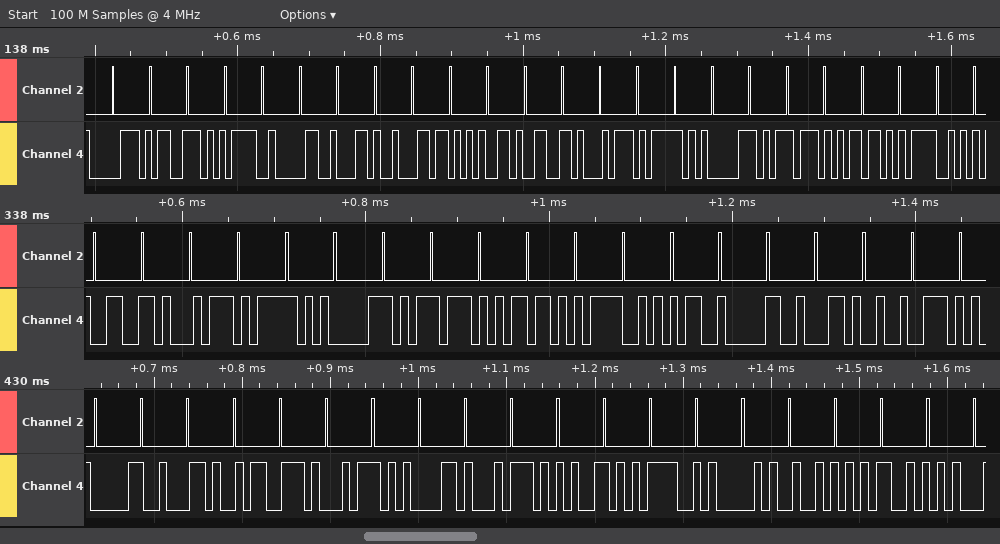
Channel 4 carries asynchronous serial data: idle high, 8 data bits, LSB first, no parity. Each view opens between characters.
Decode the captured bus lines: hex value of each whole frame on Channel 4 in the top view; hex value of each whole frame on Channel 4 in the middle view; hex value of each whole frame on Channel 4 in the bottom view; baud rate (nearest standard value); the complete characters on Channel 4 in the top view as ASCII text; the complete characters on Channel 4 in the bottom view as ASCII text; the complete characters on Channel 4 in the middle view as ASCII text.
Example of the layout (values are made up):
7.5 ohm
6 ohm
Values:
70, 73, 3D, 30, 2C, 6C, 65, 66, 74, 5F, 70, 77, 6D, 3D
66, 74, 5F, 70, 77, 6D, 3D, 35, 30, 2C, 72
30, 2C, 73, 74, 61, 74, 65, 3D, 41, 52, 4D
115200 baud
"ps=0,left_pwm="
"0,state=ARM"
"ft_pwm=50,r"
